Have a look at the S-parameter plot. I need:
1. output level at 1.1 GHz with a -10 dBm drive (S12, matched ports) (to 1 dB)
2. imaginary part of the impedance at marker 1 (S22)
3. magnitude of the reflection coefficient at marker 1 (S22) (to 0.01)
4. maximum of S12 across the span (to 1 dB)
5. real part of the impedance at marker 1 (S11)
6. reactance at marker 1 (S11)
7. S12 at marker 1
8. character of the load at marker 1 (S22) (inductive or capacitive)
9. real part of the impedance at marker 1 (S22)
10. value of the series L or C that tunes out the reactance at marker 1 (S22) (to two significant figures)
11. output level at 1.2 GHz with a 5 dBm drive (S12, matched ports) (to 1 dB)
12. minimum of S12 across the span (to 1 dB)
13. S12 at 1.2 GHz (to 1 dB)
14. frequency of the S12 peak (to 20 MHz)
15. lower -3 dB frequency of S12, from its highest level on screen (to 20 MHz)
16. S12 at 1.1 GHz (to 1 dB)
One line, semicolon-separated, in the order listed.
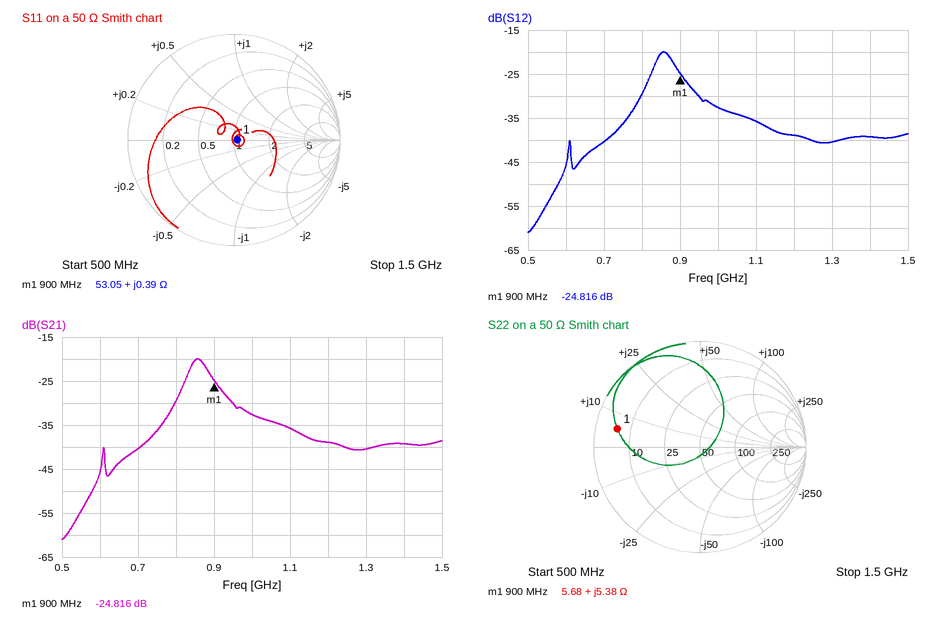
-46 dBm; +5.38 Ω; 0.80; -20 dB; 53.05 Ω; +0.39 Ω; -24.816 dB; inductive; 5.68 Ω; 33 pF; -34 dBm; -61 dB; -39 dB; 860 MHz; 840 MHz; -36 dB
